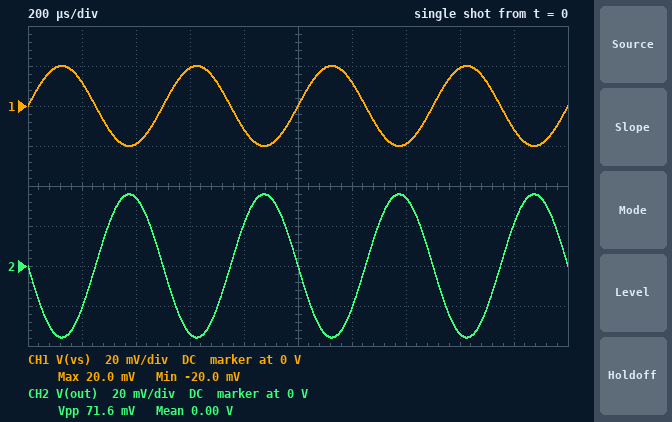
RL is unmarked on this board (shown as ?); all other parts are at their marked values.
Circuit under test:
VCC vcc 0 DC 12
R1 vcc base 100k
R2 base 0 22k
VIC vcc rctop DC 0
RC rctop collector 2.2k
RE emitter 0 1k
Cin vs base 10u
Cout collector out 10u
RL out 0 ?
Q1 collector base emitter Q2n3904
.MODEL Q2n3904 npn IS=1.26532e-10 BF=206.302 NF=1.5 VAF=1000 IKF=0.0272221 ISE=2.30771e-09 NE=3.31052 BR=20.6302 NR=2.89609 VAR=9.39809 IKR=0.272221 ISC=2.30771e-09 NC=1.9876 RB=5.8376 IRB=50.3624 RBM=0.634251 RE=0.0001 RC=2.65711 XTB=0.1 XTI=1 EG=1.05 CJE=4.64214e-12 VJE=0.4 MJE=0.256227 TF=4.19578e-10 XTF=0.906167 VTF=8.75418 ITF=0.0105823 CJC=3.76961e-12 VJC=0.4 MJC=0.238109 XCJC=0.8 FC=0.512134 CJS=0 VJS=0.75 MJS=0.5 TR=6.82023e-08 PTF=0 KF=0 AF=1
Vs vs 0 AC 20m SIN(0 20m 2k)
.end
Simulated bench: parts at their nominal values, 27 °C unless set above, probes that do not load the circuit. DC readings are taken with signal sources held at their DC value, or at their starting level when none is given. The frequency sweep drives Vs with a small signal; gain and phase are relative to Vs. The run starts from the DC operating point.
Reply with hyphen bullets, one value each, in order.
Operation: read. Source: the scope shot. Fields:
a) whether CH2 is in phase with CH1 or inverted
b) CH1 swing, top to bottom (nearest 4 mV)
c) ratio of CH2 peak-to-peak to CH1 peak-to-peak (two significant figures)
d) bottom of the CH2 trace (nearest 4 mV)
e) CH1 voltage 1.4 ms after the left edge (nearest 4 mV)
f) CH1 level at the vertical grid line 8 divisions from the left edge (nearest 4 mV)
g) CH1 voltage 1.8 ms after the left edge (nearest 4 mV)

- inverted
- 40 mV
- 1.8
- -36 mV
- -20 mV
- 20 mV
- -12 mV
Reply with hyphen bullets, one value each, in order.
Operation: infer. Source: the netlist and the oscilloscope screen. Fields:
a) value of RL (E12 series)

- 12 kΩ
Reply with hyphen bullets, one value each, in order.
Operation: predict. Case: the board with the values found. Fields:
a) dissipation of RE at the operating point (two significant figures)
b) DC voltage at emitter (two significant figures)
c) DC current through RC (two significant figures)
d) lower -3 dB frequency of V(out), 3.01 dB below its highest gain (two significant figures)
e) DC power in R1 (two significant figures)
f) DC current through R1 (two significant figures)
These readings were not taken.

- 1.8 mW
- 1.3 V
- 1.3 mA
- 1.6 Hz
- 1.0 mW
- 100 µA
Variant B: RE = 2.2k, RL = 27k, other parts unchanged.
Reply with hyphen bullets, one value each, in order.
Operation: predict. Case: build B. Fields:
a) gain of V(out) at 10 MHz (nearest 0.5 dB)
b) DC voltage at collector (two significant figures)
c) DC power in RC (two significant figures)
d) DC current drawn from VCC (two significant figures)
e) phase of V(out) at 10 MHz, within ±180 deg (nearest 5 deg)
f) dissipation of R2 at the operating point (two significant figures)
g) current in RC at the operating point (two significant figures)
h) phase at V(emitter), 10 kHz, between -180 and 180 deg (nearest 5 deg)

- -1.0 dB
- 11 V
- 940 µW
- 750 µA
- 150 deg
- 190 µW
- 650 µA
- 0 deg
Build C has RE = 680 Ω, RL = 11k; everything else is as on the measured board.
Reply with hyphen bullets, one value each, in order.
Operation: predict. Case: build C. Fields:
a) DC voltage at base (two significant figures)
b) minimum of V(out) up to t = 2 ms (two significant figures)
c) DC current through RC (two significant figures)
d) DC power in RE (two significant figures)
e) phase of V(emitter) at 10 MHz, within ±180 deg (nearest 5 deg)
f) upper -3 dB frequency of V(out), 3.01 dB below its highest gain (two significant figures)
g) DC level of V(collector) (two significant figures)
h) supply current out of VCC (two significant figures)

- 1.9 V
- -52 mV
- 1.8 mA
- 2.3 mW
- 0 deg
- 61 MHz
- 8.0 V
- 1.9 mA
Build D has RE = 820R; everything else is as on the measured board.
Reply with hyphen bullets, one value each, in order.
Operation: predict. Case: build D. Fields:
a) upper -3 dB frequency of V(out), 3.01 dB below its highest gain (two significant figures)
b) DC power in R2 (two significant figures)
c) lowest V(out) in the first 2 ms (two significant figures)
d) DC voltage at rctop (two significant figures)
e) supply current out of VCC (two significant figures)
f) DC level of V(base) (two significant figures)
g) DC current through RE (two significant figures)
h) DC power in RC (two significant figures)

- 75 MHz
- 170 µW
- -44 mV
- 12 V
- 1.7 mA
- 1.9 V
- 1.6 mA
- 5.4 mW
